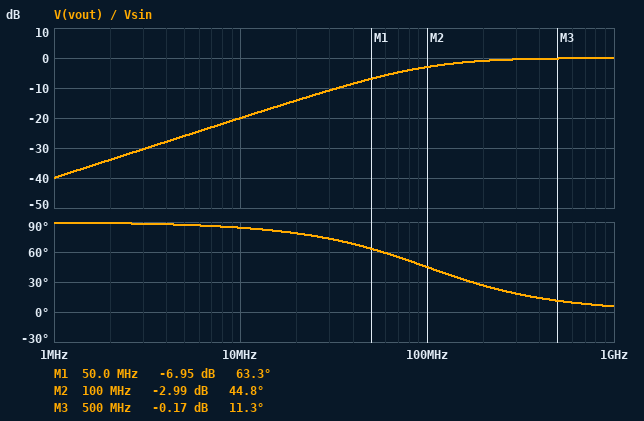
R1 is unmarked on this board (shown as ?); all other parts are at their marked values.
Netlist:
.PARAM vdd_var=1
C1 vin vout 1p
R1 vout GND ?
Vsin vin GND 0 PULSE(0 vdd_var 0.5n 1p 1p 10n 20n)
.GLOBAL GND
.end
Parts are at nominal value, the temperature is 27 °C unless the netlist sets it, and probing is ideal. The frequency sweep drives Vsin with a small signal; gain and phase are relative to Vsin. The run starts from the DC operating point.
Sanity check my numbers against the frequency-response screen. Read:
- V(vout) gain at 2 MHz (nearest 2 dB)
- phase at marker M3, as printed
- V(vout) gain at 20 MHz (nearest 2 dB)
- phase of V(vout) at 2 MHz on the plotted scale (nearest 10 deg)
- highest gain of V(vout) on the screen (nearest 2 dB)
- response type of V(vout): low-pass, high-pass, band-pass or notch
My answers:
-34 dB
11.3 deg
-14 dB
90 deg
0 dB
high-pass
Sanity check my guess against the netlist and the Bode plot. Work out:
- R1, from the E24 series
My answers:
1.6 kΩ
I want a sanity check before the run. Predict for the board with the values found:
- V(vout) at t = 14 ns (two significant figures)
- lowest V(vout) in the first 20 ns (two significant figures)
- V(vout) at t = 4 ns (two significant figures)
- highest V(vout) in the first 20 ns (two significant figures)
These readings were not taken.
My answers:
-110 mV
-1.0 V
110 mV
1.0 V
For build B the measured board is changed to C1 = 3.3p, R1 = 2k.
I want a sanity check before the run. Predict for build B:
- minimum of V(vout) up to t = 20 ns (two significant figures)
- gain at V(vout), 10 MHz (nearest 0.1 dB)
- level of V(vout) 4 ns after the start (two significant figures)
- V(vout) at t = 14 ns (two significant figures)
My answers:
-780 mV
-8.3 dB
590 mV
-460 mV
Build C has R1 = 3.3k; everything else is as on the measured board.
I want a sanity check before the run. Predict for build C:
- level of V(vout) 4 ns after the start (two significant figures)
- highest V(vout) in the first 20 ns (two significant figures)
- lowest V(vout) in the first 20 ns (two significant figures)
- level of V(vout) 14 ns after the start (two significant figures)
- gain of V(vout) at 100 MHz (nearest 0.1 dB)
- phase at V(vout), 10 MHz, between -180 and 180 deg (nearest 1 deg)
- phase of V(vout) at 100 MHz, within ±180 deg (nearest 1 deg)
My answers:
350 mV
1.0 V
-950 mV
-330 mV
-0.9 dB
78 deg
26 deg
